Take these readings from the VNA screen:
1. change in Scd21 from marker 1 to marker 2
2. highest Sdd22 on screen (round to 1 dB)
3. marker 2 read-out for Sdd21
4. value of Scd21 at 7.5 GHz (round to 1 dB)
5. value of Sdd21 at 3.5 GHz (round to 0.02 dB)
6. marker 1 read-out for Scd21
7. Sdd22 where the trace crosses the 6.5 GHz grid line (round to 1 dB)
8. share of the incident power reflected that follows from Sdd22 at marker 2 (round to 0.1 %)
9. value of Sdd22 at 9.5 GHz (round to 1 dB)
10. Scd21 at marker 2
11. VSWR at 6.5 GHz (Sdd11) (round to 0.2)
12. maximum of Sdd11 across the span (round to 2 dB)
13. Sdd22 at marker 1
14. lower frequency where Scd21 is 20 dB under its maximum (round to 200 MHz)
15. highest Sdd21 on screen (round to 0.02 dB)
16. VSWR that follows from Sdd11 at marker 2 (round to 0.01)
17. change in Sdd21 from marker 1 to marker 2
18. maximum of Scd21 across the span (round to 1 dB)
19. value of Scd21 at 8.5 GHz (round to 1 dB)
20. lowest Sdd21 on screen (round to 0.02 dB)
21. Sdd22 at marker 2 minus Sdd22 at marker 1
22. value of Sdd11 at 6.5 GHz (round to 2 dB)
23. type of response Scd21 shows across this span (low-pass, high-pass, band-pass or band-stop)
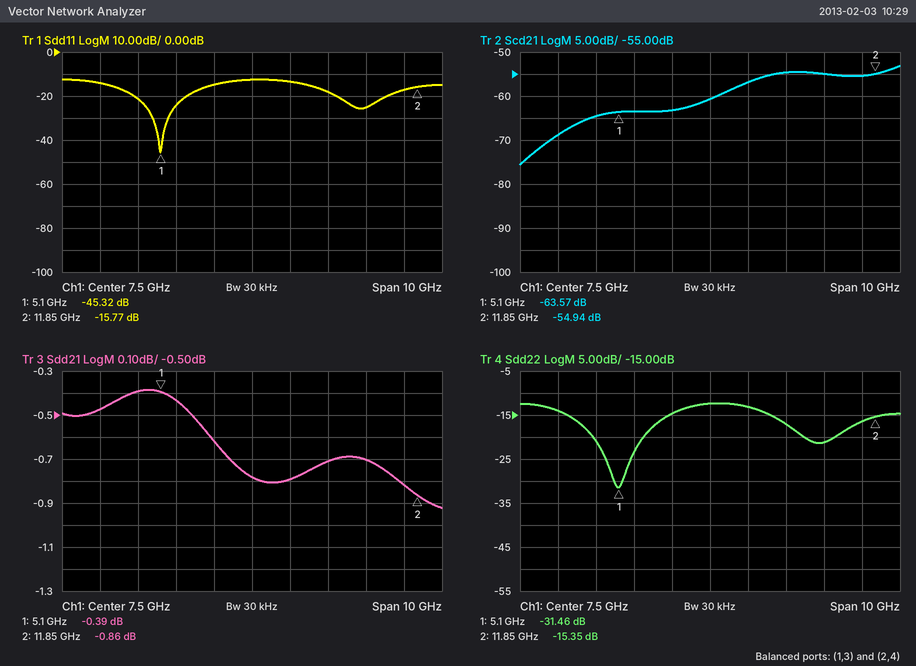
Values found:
8.63 dB
-12 dB
-0.86 dB
-61 dB
-0.48 dB
-63.57 dB
-15 dB
2.9 %
-17 dB
-54.94 dB
1.4
-12 dB
-31.46 dB
2.8 GHz
-0.38 dB
1.39
-0.47 dB
-53 dB
-57 dB
-0.92 dB
16.11 dB
-14 dB
high-pass
